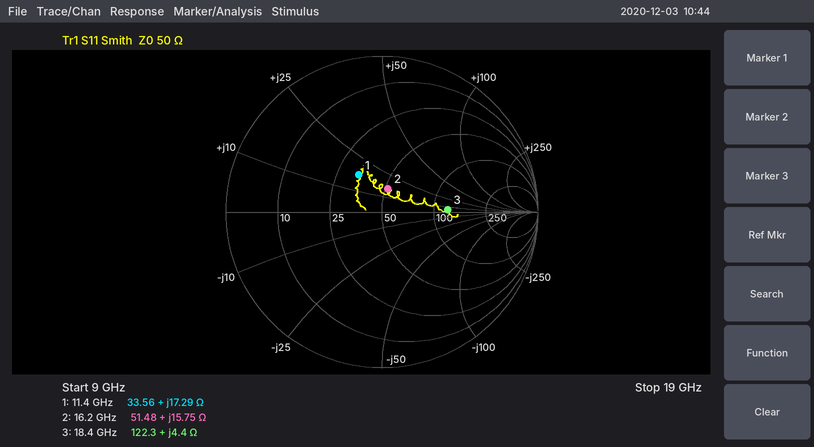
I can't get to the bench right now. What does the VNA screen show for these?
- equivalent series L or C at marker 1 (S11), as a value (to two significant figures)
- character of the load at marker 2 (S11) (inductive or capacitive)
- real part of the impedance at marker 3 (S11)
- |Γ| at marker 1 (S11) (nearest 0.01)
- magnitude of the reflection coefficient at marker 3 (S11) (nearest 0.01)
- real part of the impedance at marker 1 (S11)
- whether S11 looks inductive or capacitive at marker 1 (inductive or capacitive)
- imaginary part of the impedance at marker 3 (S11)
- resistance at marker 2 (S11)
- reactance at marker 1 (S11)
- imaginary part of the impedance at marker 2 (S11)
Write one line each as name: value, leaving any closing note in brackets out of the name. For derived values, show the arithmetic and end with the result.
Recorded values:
equivalent series L or C at marker 1 (S11), as a value: L = 17.29 Ω/(2π × 11.4 GHz) ≈ 241 pH, so 240 pH to two significant figures
character of the load at marker 2 (S11): inductive
real part of the impedance at marker 3: 122.3 Ω
|Γ| at marker 1 (S11): 0.28
magnitude of the reflection coefficient at marker 3 (S11): 0.42
real part of the impedance at marker 1: 33.56 Ω
whether S11 looks inductive or capacitive at marker 1: inductive
imaginary part of the impedance at marker 3: +4.4 Ω
resistance at marker 2: 51.48 Ω
reactance at marker 1: +17.29 Ω
imaginary part of the impedance at marker 2: +15.75 Ω
